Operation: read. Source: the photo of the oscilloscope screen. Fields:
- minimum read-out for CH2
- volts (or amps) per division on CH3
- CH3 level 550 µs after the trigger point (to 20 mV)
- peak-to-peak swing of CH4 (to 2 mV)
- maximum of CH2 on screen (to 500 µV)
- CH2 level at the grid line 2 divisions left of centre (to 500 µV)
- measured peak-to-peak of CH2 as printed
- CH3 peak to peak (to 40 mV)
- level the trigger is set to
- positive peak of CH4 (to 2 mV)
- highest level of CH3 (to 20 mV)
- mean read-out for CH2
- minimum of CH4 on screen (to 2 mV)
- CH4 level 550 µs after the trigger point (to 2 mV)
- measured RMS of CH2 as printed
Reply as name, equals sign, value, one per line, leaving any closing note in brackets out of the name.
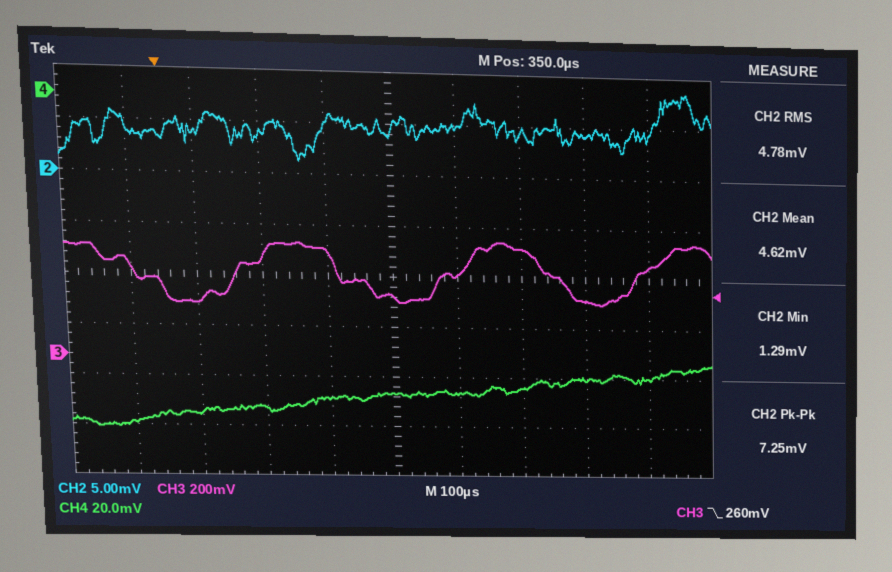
minimum read-out for CH2 = 1.29 mV
volts (or amps) per division on CH3 = 200 mV
CH3 level 550 µs after the trigger point = 440 mV
peak-to-peak swing of CH4 = 26 mV
maximum of CH2 on screen = 8.5 mV
CH2 level at the grid line 2 divisions left of centre = 4.0 mV
measured peak-to-peak of CH2 as printed = 7.25 mV
CH3 peak to peak = 240 mV
level the trigger is set to = 260 mV
positive peak of CH4 = -104 mV
highest level of CH3 = 460 mV
mean read-out for CH2 = 4.62 mV
minimum of CH4 on screen = -130 mV
CH4 level 550 µs after the trigger point = -114 mV
measured RMS of CH2 as printed = 4.78 mV
